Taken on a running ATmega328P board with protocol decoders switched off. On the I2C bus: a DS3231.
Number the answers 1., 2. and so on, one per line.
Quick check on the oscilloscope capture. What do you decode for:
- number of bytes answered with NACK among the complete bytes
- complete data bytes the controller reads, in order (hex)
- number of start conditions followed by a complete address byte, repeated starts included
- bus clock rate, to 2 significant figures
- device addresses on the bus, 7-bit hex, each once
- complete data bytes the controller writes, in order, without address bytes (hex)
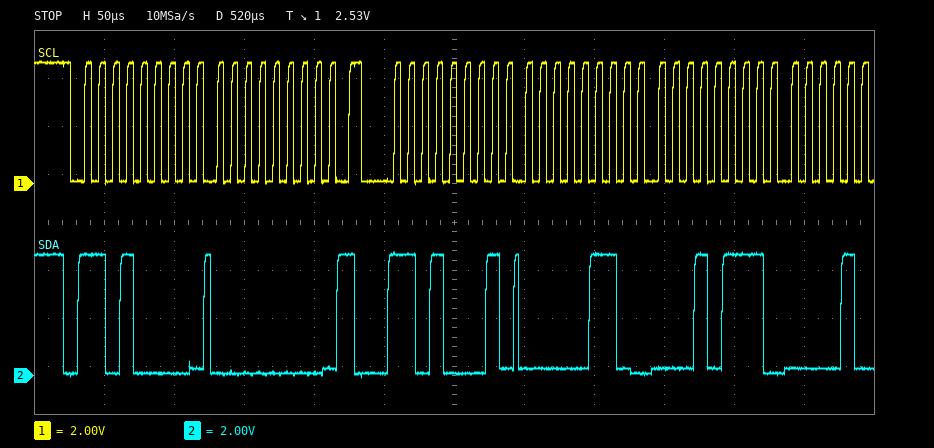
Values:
1. 0
2. 06 17
3. 2
4. 100 kHz
5. 0x68
6. 00
